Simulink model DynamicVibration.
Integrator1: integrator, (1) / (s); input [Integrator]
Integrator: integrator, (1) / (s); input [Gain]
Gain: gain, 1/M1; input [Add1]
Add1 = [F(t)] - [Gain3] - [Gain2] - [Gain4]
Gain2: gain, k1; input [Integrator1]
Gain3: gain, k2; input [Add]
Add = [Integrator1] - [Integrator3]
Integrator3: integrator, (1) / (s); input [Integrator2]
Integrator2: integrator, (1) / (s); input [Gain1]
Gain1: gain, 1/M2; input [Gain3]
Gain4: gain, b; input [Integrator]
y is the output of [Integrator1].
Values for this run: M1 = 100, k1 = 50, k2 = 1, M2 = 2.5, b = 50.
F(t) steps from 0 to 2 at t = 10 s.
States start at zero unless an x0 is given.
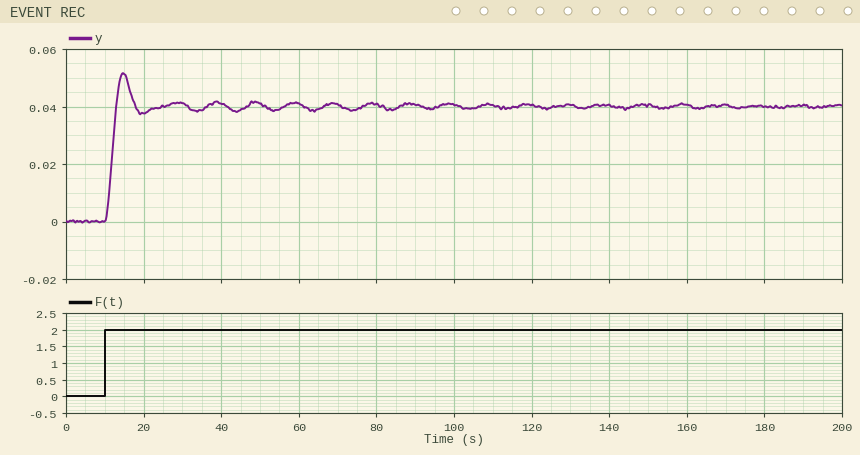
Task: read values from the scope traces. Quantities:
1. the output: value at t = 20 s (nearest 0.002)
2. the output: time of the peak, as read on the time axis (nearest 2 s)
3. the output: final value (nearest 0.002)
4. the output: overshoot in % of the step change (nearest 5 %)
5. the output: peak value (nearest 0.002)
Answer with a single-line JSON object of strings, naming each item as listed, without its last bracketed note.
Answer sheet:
{"the output: value at t = 20 s": "0.038", "the output: time of the peak, as read on the time axis": "14 s", "the output: final value": "0.040", "the output: overshoot in % of the step change": "30 %", "the output: peak value": "0.052"}
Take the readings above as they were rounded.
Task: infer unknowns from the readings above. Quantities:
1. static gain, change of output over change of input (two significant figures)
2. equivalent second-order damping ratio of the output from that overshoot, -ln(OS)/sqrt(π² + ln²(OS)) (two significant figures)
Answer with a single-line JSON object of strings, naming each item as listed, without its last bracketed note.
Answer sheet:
{"static gain, change of output over change of input": "0.020", "equivalent second-order damping ratio of the output from that overshoot, -ln(OS)/sqrt(π² + ln²(OS))": "0.36"}
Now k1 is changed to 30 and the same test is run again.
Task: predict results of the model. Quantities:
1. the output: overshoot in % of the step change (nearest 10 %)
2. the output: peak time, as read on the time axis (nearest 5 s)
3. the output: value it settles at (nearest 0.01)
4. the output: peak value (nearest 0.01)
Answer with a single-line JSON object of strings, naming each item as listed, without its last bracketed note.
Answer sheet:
{"the output: overshoot in % of the step change": "20 %", "the output: peak time, as read on the time axis": "15 s", "the output: value it settles at": "0.07", "the output: peak value": "0.08"}
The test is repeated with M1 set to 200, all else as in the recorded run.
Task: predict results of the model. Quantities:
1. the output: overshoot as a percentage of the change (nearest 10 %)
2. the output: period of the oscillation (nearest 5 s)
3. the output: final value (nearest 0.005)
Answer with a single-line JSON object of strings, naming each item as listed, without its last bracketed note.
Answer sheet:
{"the output: overshoot as a percentage of the change": "40 %", "the output: period of the oscillation": "15 s", "the output: final value": "0.040"}
